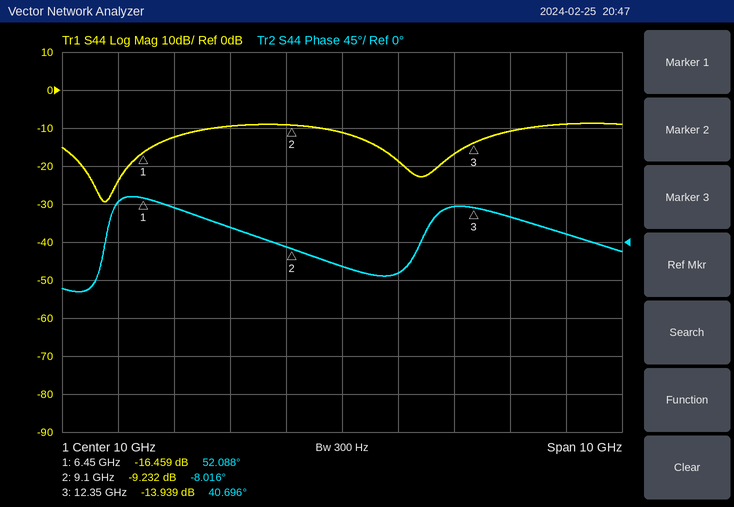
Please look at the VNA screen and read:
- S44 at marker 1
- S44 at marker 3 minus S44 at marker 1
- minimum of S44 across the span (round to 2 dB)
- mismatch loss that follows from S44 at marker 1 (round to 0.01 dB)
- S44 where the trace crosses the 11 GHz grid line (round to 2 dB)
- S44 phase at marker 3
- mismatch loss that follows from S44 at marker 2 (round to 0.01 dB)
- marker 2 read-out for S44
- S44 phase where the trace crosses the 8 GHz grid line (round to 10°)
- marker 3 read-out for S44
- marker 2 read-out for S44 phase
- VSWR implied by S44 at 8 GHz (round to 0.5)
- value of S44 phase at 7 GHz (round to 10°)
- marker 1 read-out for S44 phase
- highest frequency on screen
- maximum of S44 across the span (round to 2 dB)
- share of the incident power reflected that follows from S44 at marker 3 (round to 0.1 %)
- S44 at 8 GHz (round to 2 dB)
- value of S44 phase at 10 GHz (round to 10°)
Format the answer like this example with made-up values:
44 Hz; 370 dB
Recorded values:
-16.459 dB; 2.520 dB; -30 dB; 0.10 dB; -18 dB; 40.696°; 0.55 dB; -9.232 dB; 20°; -13.939 dB; -8.016°; 2.0; 40°; 52.088°; 15 GHz; -8 dB; 4.0 %; -10 dB; -30°
